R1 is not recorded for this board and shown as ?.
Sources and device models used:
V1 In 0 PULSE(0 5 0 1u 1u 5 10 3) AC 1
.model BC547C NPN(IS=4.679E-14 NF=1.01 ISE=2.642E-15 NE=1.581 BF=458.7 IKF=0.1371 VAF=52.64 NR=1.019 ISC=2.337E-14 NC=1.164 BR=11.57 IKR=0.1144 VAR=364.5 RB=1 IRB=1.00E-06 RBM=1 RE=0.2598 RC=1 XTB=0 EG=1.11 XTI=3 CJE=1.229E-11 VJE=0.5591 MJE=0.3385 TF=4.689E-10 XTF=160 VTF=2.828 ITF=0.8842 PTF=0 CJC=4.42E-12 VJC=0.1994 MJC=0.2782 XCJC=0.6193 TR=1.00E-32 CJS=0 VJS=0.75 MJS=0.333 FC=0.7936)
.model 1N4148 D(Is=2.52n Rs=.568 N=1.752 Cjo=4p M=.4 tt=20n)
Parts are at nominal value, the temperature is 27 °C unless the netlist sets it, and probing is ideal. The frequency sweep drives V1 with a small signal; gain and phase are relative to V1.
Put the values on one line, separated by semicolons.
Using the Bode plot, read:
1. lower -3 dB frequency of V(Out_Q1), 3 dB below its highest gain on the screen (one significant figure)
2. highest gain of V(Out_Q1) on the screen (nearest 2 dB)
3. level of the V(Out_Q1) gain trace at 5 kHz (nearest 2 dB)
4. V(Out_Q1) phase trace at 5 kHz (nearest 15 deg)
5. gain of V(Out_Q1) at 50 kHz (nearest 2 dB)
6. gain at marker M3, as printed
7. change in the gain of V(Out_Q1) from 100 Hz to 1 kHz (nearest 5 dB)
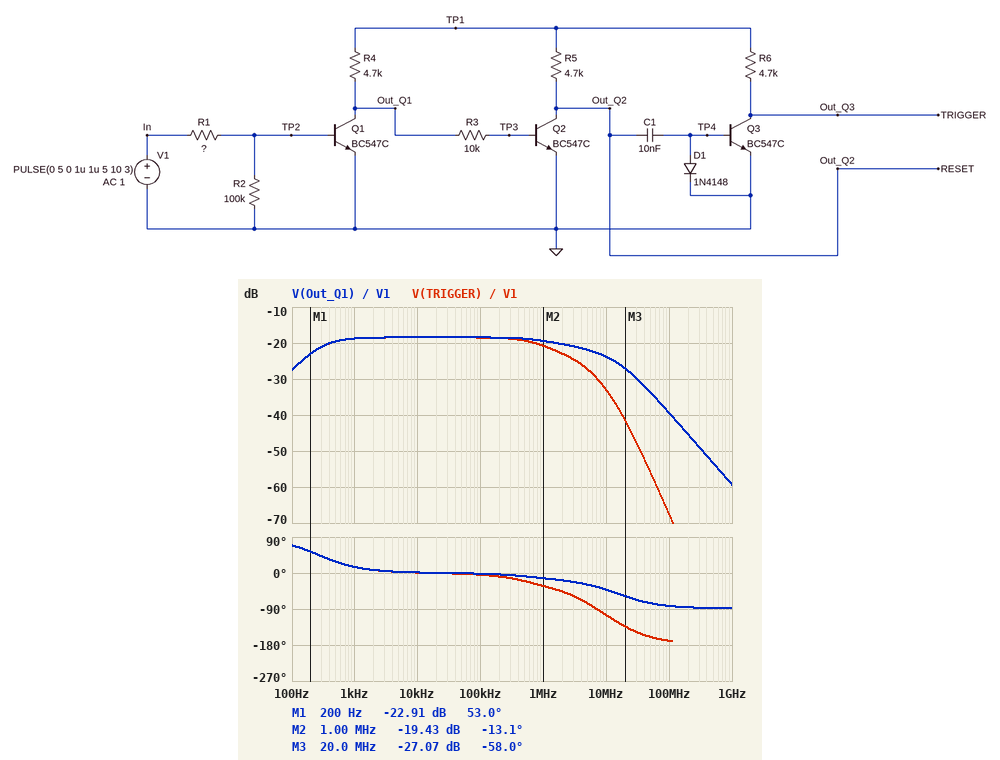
300 Hz; -18 dB; -18 dB; 0 deg; -18 dB; -27.07 dB; 10 dB
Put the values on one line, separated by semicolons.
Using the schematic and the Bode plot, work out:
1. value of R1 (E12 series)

12 kΩ
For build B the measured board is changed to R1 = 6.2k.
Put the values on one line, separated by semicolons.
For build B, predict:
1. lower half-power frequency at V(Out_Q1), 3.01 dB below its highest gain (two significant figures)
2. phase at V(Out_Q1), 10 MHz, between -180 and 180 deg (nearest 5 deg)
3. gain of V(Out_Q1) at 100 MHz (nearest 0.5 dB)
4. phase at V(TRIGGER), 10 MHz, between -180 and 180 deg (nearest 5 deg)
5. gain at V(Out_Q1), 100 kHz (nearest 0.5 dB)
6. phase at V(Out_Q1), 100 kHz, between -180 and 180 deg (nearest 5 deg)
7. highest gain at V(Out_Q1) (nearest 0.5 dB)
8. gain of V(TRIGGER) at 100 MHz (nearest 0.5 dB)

500 Hz; -35 deg; -33.5 dB; -100 deg; -18.0 dB; 0 deg; -16.0 dB; -62.0 dB
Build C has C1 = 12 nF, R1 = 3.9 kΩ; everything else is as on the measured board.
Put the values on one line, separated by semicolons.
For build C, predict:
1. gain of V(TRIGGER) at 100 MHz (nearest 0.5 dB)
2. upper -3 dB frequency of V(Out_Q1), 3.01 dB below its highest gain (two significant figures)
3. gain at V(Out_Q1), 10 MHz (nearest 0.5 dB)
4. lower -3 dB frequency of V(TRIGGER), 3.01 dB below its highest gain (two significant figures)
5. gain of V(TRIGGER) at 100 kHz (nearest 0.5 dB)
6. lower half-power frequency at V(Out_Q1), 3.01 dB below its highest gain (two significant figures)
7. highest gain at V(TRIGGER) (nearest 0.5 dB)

-58.0 dB; 16 MHz; -14.5 dB; 350 Hz; -18.0 dB; 870 kHz; -17.0 dB
